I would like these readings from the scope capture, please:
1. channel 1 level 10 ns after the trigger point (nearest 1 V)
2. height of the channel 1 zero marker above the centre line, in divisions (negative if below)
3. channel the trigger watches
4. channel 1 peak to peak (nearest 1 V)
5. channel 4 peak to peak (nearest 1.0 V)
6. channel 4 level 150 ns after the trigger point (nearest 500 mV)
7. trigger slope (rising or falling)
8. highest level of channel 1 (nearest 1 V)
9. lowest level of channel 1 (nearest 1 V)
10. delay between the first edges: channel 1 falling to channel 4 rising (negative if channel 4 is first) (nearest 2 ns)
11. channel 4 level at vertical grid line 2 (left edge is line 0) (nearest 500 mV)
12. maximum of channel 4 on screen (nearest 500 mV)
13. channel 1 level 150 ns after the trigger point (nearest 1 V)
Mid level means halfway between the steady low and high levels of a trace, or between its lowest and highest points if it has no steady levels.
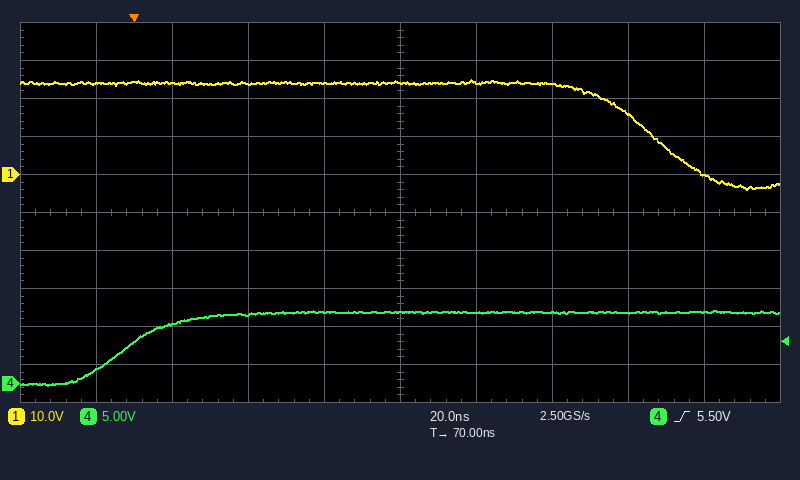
24 V
+1.0 div
channel 4
29 V
10.0 V
9.5 V
rising
25 V
-4 V
-138 ns
8.0 V
9.5 V
0 V
